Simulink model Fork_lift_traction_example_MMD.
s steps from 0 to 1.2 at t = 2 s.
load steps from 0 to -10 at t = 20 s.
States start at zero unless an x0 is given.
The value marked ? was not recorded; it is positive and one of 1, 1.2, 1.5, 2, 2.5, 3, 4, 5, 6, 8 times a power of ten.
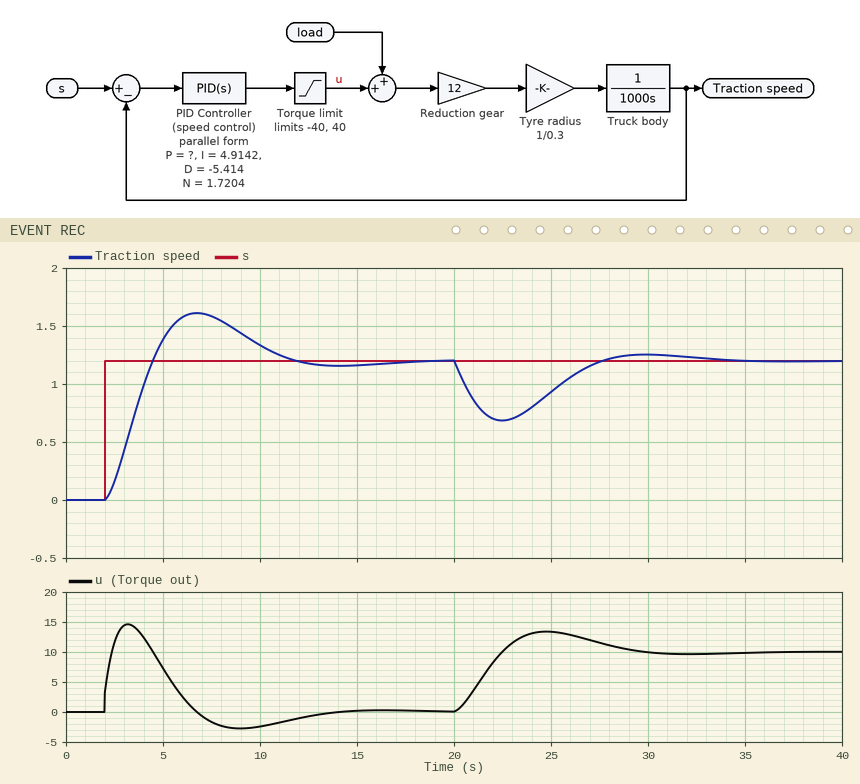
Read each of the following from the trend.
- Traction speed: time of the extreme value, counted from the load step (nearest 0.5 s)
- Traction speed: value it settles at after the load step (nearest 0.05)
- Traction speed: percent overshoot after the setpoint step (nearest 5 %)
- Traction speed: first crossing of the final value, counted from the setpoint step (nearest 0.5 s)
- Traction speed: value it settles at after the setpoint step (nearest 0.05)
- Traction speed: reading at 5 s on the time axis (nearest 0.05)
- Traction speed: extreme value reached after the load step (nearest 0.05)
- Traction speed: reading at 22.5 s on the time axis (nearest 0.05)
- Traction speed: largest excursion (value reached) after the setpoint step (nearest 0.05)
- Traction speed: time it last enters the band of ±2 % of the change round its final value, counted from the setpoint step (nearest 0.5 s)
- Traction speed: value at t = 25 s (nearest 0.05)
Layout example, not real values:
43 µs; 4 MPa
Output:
2.5 s; 1.20; 35 %; 2.5 s; 1.20; 1.40; 0.70; 0.70; 1.60; 14.5 s; 0.95
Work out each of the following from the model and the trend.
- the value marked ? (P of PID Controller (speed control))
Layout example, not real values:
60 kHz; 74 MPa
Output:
12
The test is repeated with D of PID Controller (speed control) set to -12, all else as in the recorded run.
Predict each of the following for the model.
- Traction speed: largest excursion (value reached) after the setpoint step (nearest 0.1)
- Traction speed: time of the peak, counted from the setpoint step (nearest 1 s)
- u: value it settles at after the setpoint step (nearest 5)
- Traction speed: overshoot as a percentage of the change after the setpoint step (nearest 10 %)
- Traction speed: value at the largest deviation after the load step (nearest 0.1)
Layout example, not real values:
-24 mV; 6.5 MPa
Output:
1.8; 4 s; 0; 50 %; 0.6
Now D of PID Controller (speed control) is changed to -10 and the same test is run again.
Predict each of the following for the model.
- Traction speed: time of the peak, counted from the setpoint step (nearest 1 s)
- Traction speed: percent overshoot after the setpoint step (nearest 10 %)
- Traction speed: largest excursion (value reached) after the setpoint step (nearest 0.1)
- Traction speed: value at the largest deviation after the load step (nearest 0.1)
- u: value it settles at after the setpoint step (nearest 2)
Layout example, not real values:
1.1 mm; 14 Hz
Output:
4 s; 40 %; 1.7; 0.6; 0
